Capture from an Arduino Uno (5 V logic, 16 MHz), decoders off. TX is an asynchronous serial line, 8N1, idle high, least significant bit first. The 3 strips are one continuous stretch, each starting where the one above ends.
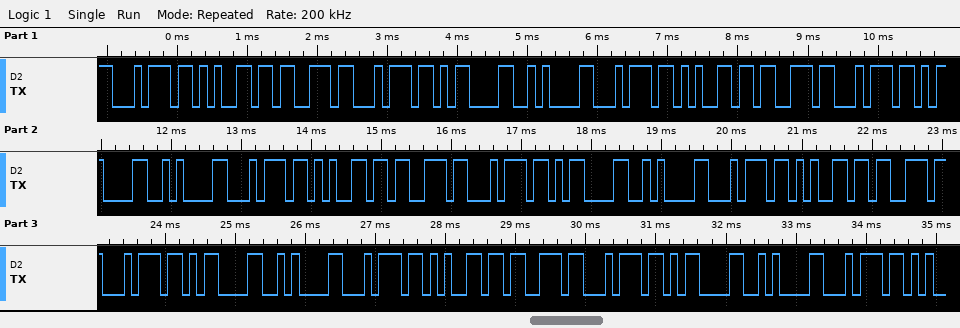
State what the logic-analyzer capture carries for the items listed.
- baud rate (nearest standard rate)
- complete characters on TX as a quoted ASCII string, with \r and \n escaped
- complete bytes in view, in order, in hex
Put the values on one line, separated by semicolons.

9600 baud; "test\r\ntest\r\ntest\r\ntest\r\ntest\r\nt"; 74 65 73 74 0D 0A 74 65 73 74 0D 0A 74 65 73 74 0D 0A 74 65 73 74 0D 0A 74 65 73 74 0D 0A 74
